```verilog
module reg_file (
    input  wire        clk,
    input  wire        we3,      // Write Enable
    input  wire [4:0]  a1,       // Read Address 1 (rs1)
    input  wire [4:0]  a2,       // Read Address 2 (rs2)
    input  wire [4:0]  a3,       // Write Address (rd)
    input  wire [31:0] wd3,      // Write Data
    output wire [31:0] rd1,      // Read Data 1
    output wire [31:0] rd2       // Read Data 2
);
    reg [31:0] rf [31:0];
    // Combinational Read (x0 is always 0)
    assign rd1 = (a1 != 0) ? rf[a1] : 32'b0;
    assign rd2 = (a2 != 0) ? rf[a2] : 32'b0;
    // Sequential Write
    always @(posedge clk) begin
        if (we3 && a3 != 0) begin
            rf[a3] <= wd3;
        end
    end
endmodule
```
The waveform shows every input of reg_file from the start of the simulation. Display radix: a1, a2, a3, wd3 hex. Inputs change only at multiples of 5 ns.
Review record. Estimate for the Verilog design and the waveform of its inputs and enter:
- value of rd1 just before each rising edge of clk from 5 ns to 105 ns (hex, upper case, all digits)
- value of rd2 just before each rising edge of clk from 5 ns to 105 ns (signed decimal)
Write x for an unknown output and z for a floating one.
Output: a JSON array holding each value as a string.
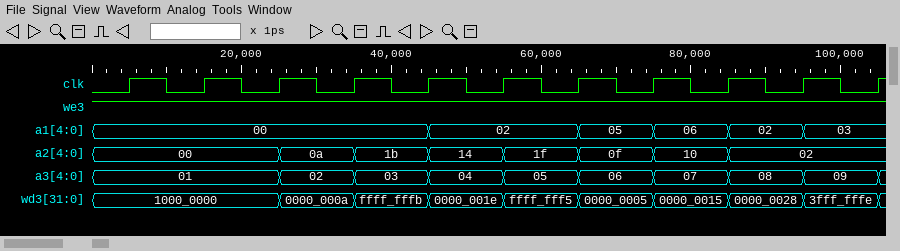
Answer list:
["00000000, 00000000, 00000000, 00000000, 00000000, 0000000A, 0000000A, FFFFFFF5, 00000005, 0000000A, FFFFFFFB", "0, 0, 0, x, x, x, x, x, x, 10, 10"]
